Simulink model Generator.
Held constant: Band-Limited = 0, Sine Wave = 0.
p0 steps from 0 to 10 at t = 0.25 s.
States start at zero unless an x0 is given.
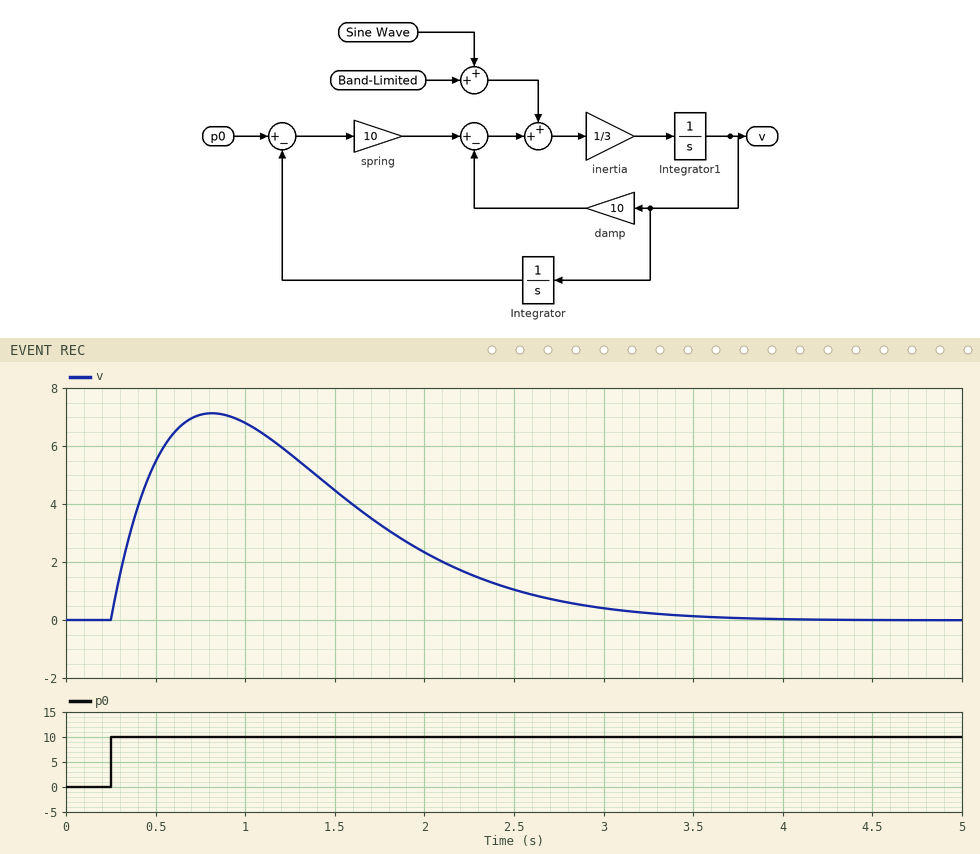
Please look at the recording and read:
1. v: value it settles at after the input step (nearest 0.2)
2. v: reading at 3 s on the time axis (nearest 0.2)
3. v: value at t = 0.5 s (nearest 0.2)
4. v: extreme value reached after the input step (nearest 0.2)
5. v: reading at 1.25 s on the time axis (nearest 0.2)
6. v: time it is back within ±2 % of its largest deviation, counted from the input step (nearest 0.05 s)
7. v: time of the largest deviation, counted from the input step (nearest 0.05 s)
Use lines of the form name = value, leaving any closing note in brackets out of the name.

v: value it settles at after the input step = 0.0
v: reading at 3 s on the time axis = 0.4
v: value at t = 0.5 s = 5.4
v: extreme value reached after the input step = 7.2
v: reading at 1.25 s on the time axis = 5.8
v: time it is back within ±2 % of its largest deviation, counted from the input step = 3.20 s
v: time of the largest deviation, counted from the input step = 0.55 s
